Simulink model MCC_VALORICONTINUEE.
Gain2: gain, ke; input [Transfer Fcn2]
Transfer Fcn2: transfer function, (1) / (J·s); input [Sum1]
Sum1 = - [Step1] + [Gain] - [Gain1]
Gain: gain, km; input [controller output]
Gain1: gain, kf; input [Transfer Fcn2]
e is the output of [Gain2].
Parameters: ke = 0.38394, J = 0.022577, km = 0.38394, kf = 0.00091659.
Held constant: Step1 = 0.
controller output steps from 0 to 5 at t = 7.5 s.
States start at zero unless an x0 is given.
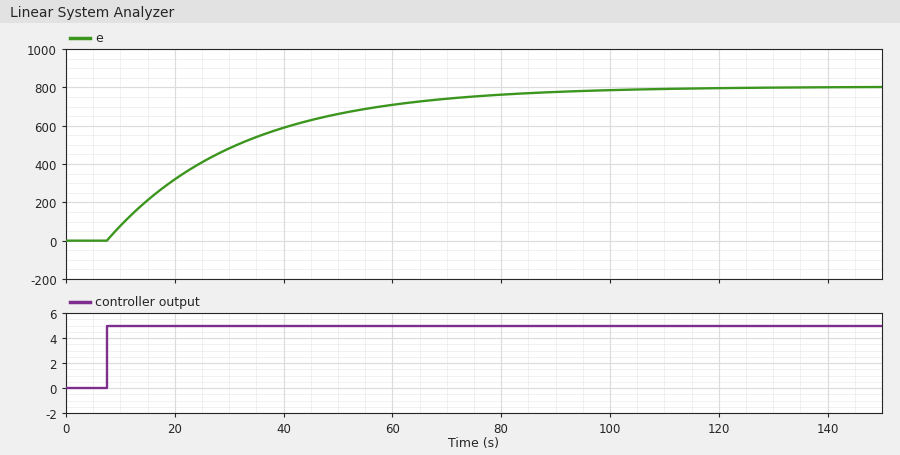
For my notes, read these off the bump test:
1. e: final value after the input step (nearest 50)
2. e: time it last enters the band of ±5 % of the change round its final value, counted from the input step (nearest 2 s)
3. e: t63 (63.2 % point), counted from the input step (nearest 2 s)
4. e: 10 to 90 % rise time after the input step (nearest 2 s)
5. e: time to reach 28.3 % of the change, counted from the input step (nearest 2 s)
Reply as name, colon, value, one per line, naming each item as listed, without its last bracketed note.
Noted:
e: final value after the input step: 800
e: time it last enters the band of ±5 % of the change round its final value, counted from the input step: 74 s
e: t63 (63.2 % point), counted from the input step: 24 s
e: 10 to 90 % rise time after the input step: 54 s
e: time to reach 28.3 % of the change, counted from the input step: 8 s
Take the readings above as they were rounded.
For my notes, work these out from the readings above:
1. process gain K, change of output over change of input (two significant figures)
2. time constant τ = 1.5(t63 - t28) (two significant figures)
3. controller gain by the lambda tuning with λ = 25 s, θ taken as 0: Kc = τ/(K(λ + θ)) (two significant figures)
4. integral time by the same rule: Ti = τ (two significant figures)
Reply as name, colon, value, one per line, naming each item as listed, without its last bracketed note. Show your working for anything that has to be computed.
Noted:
process gain K, change of output over change of input: (800 - 0) / 5 = 160
time constant τ = 1.5(t63 - t28): 1.5 × (24 - 8) = 24 s
controller gain by the lambda tuning with λ = 25 s, θ taken as 0: Kc = τ/(K(λ + θ)): 24 / (160 × (25 + 0)) = 0.0060
integral time by the same rule: Ti = τ: 24 s
